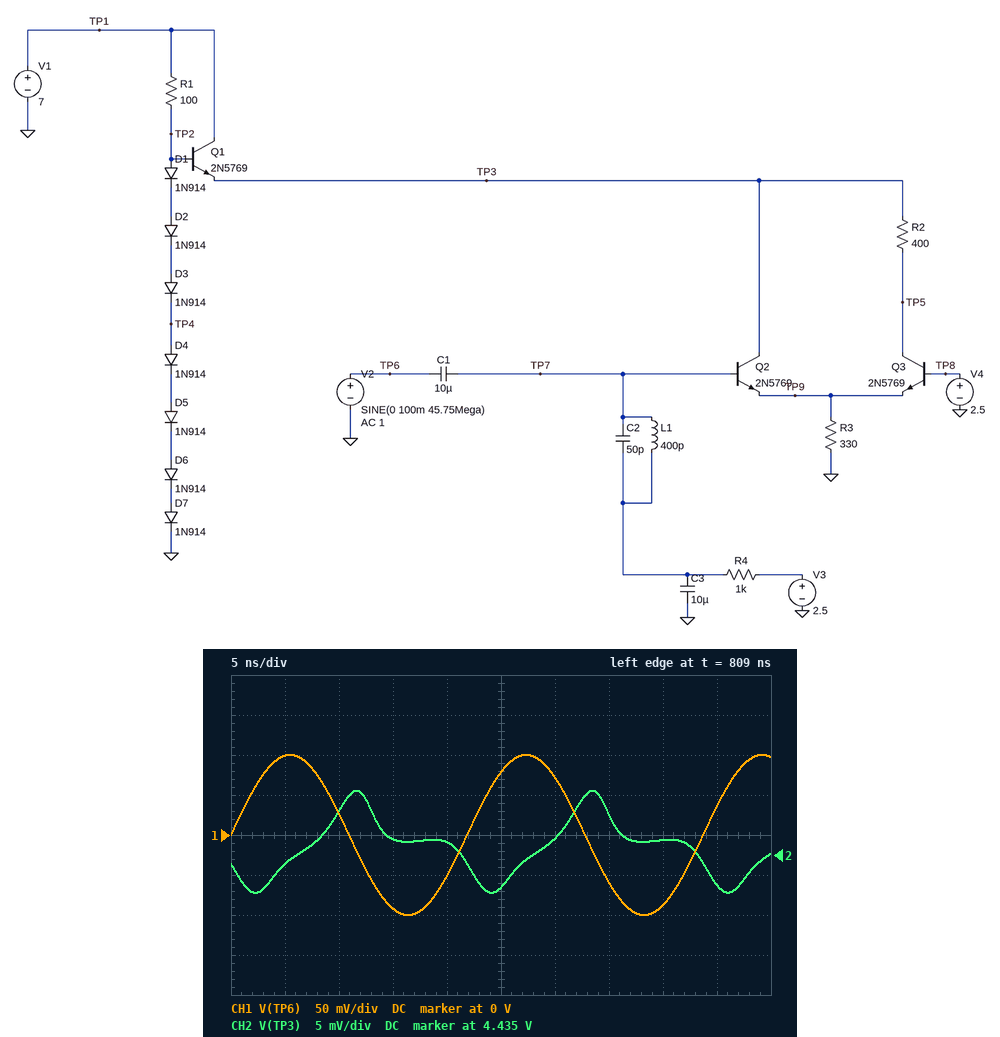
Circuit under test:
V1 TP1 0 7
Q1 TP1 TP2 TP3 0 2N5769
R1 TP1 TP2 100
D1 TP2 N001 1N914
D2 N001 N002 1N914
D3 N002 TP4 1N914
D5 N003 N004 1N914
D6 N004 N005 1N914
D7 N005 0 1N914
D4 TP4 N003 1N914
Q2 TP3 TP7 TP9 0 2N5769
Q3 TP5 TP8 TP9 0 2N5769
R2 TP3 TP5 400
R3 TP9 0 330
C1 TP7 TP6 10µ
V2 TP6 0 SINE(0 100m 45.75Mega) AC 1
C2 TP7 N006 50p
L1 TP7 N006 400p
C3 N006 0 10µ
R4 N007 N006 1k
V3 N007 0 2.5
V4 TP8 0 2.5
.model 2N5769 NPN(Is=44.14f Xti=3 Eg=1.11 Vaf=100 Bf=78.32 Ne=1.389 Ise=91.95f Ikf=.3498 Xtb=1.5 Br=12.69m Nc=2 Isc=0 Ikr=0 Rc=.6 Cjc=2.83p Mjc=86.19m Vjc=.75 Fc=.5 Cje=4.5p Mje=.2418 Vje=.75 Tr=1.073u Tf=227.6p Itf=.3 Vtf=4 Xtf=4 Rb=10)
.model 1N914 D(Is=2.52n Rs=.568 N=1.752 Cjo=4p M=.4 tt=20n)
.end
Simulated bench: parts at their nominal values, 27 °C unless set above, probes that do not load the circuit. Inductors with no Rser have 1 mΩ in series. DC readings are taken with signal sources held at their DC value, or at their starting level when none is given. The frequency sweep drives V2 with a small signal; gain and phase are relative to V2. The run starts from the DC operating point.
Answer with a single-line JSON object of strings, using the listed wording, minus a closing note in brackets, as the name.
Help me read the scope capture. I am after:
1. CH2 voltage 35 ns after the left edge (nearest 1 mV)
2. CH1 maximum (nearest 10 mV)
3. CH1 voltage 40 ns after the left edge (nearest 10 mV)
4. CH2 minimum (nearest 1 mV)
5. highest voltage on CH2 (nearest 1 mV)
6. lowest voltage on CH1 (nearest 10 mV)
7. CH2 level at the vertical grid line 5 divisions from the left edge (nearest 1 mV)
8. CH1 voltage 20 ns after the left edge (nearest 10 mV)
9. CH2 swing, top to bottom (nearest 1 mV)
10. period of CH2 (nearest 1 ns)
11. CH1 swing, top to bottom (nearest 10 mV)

{"CH2 voltage 35 ns after the left edge": "4.440 V", "CH1 maximum": "100 mV", "CH1 voltage 40 ns after the left edge": "-90 mV", "CH2 minimum": "4.430 V", "highest voltage on CH2": "4.443 V", "lowest voltage on CH1": "-100 mV", "CH2 level at the vertical grid line 5 divisions from the left edge": "4.431 V", "CH1 voltage 20 ns after the left edge": "-50 mV", "CH2 swing, top to bottom": "13 mV", "period of CH2": "22 ns", "CH1 swing, top to bottom": "200 mV"}
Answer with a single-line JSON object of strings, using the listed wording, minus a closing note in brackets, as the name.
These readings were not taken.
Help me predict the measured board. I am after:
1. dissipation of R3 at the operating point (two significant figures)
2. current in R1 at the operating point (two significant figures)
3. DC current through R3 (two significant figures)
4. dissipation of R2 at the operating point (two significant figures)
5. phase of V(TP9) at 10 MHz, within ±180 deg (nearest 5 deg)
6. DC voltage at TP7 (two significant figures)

{"dissipation of R3 at the operating point": "10 mW", "current in R1 at the operating point": "19 mA", "DC current through R3": "5.6 mA", "dissipation of R2 at the operating point": "6.1 mW", "phase of V(TP9) at 10 MHz, within ±180 deg": "5 deg", "DC voltage at TP7": "2.5 V"}
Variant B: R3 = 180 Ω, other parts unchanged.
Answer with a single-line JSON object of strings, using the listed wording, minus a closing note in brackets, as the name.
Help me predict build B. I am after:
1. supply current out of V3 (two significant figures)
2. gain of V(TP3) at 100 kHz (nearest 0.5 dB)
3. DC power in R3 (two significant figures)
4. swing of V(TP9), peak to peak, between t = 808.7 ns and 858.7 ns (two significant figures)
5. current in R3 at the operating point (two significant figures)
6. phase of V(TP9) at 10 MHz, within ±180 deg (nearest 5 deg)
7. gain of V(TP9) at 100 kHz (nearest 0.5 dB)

{"supply current out of V3": "39 µA", "gain of V(TP3) at 100 kHz": "-23.0 dB", "DC power in R3": "18 mW", "swing of V(TP9), peak to peak, between t = 808.7 ns and 858.7 ns": "100 mV", "current in R3 at the operating point": "10 mA", "phase of V(TP9) at 10 MHz, within ±180 deg": "0 deg", "gain of V(TP9) at 100 kHz": "-11.0 dB"}
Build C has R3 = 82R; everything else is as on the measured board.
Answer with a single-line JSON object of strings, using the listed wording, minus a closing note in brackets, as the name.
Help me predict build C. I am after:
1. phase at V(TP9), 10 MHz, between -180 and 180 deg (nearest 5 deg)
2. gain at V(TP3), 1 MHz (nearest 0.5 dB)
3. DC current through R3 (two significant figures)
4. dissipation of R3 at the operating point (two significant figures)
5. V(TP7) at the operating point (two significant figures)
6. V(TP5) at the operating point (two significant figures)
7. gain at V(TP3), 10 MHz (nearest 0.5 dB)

{"phase at V(TP9), 10 MHz, between -180 and 180 deg": "0 deg", "gain at V(TP3), 1 MHz": "-22.5 dB", "DC current through R3": "21 mA", "dissipation of R3 at the operating point": "37 mW", "V(TP7) at the operating point": "2.4 V", "V(TP5) at the operating point": "1.9 V", "gain at V(TP3), 10 MHz": "-15.0 dB"}
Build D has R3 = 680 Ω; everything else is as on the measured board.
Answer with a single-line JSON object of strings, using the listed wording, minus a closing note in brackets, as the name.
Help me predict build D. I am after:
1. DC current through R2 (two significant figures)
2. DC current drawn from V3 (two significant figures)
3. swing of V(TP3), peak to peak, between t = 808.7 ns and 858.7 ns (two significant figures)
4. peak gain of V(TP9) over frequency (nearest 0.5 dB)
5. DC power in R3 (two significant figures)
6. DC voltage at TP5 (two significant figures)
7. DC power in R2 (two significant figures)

{"DC current through R2": "1.7 mA", "DC current drawn from V3": "15 µA", "swing of V(TP3), peak to peak, between t = 808.7 ns and 858.7 ns": "11 mV", "peak gain of V(TP9) over frequency": "4.5 dB", "DC power in R3": "5.1 mW", "DC voltage at TP5": "3.8 V", "DC power in R2": "1.2 mW"}
